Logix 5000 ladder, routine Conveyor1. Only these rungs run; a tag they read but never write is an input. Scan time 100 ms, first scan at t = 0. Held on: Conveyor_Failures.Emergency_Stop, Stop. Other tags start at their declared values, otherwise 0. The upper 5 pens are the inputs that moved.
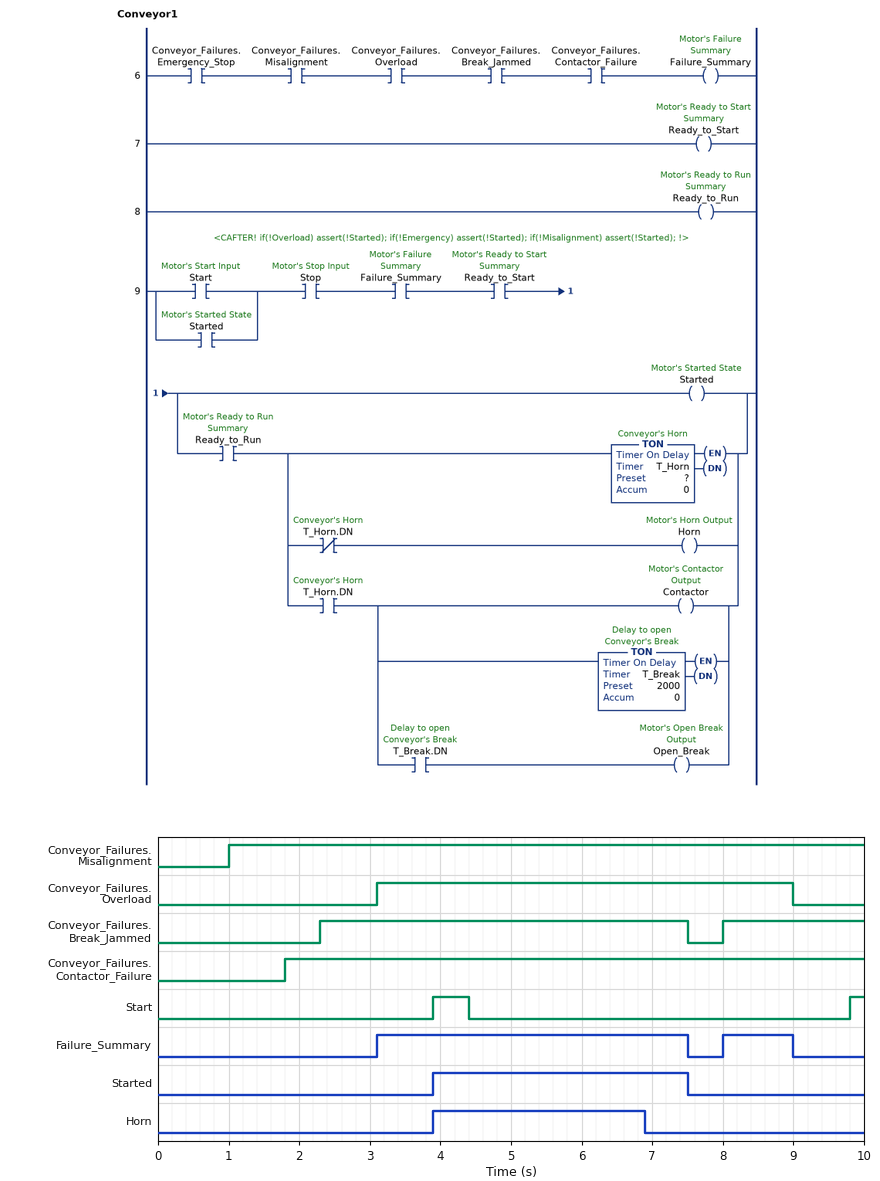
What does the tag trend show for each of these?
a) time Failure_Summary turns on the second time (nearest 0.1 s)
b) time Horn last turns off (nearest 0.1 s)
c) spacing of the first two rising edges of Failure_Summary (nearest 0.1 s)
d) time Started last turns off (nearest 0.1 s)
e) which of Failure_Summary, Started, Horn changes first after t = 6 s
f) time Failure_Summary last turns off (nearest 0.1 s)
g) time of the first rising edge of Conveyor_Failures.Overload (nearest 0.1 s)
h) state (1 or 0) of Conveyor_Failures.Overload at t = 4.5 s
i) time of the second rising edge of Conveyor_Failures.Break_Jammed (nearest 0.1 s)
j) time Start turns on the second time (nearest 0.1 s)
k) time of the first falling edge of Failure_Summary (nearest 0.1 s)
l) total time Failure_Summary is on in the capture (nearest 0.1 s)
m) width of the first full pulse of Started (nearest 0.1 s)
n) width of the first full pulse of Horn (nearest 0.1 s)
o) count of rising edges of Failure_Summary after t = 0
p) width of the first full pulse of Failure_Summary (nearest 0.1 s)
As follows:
8.0 s
6.9 s
4.9 s
7.5 s
Horn
9.0 s
3.1 s
1
8.0 s
9.8 s
7.5 s
5.4 s
3.6 s
3.0 s
2
4.4 s
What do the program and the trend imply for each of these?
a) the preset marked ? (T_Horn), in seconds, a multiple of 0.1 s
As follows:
3.0 s
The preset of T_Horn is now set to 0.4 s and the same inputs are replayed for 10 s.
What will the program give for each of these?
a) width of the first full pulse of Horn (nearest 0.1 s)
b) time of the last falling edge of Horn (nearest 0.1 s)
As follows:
0.4 s
4.3 s
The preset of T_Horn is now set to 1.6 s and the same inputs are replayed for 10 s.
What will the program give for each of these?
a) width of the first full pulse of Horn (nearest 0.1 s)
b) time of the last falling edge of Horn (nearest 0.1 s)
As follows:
1.6 s
5.5 s
